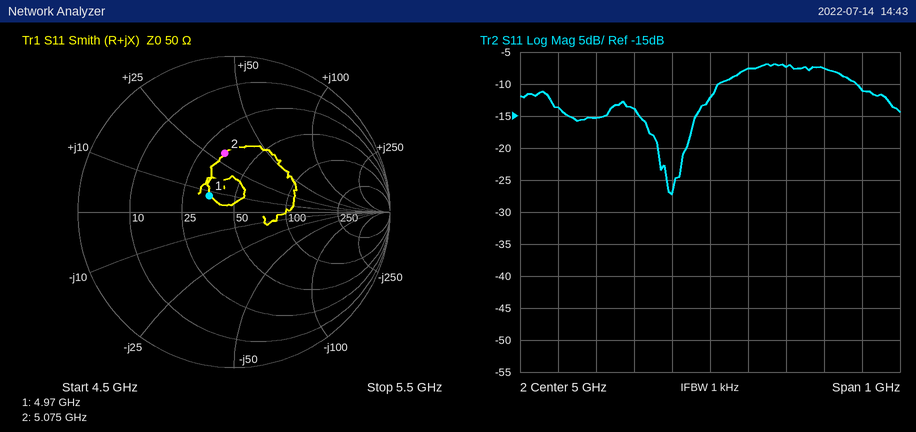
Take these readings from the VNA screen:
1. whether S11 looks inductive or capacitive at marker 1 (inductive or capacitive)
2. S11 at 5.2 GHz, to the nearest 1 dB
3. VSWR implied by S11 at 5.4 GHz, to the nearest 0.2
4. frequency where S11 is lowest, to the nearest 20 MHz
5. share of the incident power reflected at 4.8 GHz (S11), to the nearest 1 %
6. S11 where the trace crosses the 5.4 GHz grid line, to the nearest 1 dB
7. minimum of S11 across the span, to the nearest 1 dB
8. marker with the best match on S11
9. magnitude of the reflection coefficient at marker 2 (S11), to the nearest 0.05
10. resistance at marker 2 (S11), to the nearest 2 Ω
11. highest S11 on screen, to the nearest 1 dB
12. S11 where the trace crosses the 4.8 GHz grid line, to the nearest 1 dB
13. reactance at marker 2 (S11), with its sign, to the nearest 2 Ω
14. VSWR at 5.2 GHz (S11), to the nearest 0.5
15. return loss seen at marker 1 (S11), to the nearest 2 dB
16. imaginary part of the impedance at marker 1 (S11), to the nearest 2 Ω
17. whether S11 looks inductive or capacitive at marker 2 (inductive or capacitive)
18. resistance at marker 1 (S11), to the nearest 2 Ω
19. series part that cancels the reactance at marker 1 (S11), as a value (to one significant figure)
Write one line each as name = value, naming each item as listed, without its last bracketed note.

whether S11 looks inductive or capacitive at marker 1 = inductive
S11 at 5.2 GHz, to the nearest 1 dB = -7 dB
VSWR implied by S11 at 5.4 GHz, to the nearest 0.2 = 1.8
frequency where S11 is lowest, to the nearest 20 MHz = 4.90 GHz
share of the incident power reflected at 4.8 GHz (S11), to the nearest 1 % = 4 %
S11 where the trace crosses the 5.4 GHz grid line, to the nearest 1 dB = -11 dB
minimum of S11 across the span, to the nearest 1 dB = -27 dB
marker with the best match on S11 = marker 1
magnitude of the reflection coefficient at marker 2 (S11), to the nearest 0.05 = 0.40
resistance at marker 2 (S11), to the nearest 2 Ω = 34 Ω
highest S11 on screen, to the nearest 1 dB = -7 dB
S11 where the trace crosses the 4.8 GHz grid line, to the nearest 1 dB = -14 dB
reactance at marker 2 (S11), with its sign, to the nearest 2 Ω = +30 Ω
VSWR at 5.2 GHz (S11), to the nearest 0.5 = 2.5
return loss seen at marker 1 (S11), to the nearest 2 dB = 14 dB
imaginary part of the impedance at marker 1 (S11), to the nearest 2 Ω = +8 Ω
whether S11 looks inductive or capacitive at marker 2 = inductive
resistance at marker 1 (S11), to the nearest 2 Ω = 36 Ω
series part that cancels the reactance at marker 1 (S11), as a value = 4 pF
